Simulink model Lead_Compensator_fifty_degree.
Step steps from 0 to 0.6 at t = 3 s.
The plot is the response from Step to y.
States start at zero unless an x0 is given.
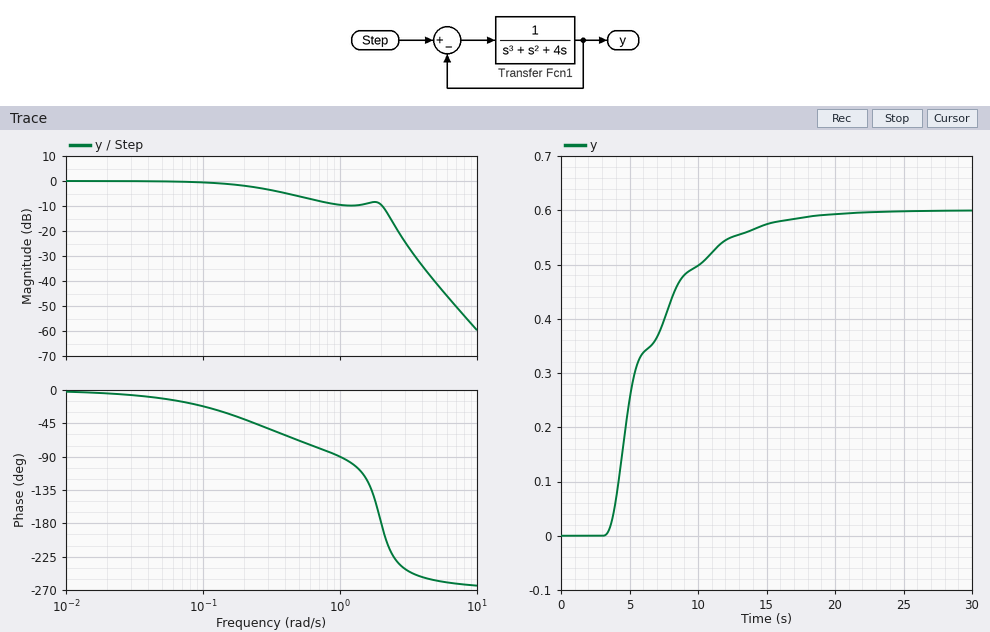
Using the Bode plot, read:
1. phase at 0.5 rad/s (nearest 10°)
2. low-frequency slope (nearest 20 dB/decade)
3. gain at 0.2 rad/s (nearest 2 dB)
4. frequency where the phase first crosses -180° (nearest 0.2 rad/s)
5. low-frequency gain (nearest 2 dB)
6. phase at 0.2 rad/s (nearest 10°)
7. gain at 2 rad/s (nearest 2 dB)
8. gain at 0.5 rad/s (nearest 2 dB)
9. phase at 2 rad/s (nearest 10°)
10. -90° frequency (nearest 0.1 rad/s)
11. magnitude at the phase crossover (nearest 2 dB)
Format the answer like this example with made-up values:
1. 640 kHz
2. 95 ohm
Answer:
1. -70°
2. 0 dB/decade
3. -2 dB
4. 2.0 rad/s
5. 0 dB
6. -40°
7. -10 dB
8. -6 dB
9. -180°
10. 1.0 rad/s
11. -10 dB
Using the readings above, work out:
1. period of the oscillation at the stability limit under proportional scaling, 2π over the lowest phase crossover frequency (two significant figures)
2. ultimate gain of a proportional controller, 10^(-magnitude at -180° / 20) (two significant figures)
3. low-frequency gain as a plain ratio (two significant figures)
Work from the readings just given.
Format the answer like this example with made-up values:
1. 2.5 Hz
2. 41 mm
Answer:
1. 3.1 s
2. 3.2
3. 1.0
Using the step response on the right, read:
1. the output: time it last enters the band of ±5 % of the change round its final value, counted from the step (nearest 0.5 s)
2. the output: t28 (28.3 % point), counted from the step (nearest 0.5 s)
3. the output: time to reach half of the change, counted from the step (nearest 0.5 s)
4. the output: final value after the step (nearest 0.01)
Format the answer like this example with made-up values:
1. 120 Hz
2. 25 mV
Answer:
1. 11.5 s
2. 1.5 s
3. 2.5 s
4. 0.60
